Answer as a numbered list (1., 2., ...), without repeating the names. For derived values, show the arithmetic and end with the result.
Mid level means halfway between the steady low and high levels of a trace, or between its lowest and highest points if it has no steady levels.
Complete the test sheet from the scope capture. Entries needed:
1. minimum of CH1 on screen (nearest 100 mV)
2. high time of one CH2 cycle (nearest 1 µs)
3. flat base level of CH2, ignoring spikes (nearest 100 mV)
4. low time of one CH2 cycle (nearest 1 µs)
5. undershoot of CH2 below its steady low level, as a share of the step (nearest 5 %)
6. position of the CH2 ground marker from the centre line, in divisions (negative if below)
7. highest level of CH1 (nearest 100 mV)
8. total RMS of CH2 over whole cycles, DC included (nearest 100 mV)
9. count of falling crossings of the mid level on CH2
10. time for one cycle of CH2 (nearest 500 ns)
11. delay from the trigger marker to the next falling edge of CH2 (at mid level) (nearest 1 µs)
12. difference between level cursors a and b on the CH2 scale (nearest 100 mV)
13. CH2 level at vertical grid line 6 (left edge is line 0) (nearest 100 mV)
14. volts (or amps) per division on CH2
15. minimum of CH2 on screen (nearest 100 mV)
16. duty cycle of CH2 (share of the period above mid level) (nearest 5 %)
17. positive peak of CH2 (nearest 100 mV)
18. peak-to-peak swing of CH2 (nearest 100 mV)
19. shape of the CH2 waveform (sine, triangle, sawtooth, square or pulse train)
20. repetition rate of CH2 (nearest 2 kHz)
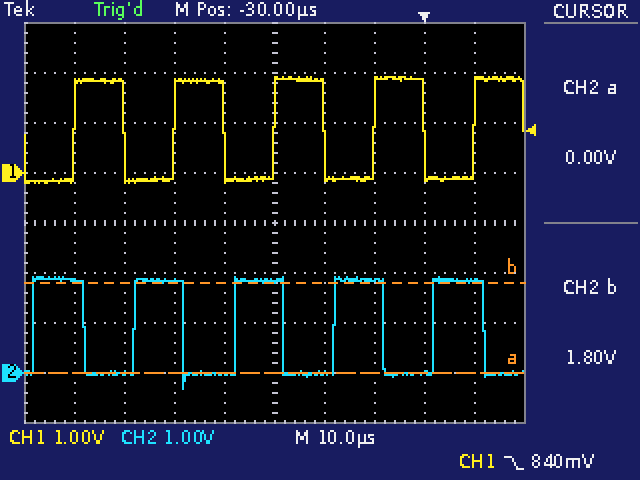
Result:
1. -200 mV
2. 10 µs
3. 0.0 V
4. 10 µs
5. 15 %
6. -3.0 div
7. 1.9 V
8. √(0.5 × (1.9 V)² + 0.5 × (0.0 V)²) ≈ 1.3 V
9. 5
10. 20.0 µs
11. 12 µs
12. 1.8 V
13. 0.0 V
14. 1 V
15. -300 mV
16. 10 µs / 20.0 µs ≈ 50 %
17. 1.9 V
18. 1.9 V − (-300 mV) = 2.2 V
19. square
20. 1 / 20.0 µs ≈ 50 kHz
